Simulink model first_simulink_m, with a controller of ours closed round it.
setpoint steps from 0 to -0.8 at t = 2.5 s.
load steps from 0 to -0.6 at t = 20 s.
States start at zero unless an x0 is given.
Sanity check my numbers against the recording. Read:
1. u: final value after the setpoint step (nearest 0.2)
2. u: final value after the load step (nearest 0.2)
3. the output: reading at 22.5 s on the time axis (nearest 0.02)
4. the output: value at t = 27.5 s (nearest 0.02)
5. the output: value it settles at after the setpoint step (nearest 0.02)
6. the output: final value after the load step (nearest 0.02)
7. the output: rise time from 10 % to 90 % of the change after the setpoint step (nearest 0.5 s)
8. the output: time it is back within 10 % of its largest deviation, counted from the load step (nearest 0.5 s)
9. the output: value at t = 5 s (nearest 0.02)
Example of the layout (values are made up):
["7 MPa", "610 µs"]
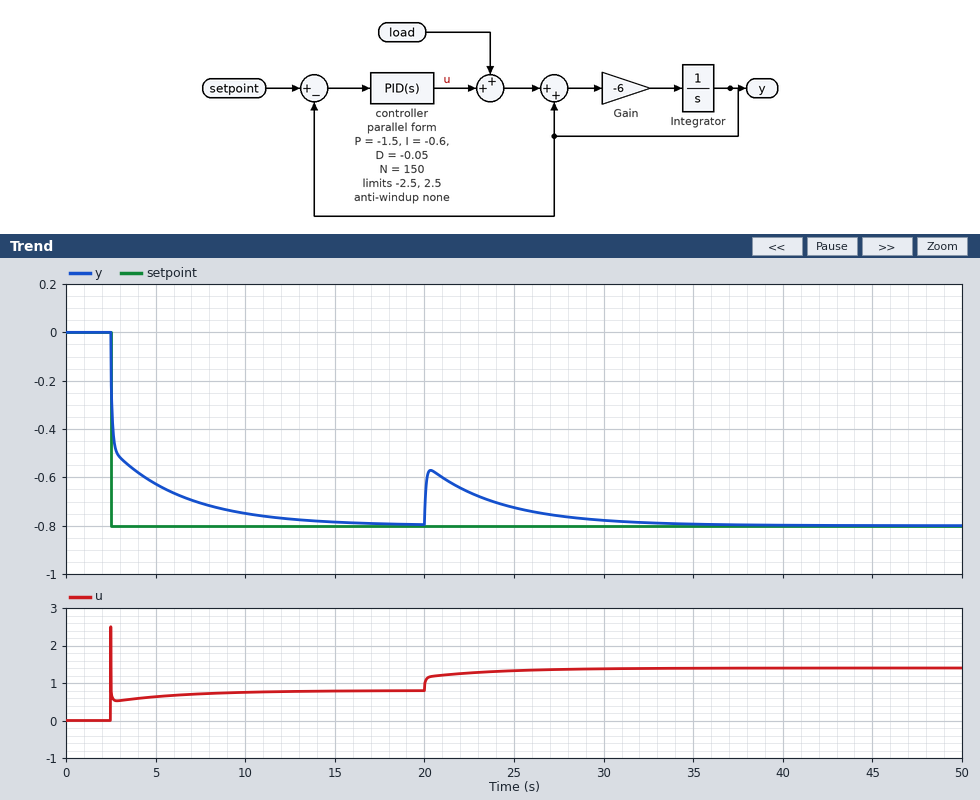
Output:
["0.8", "1.4", "-0.66", "-0.76", "-0.80", "-0.80", "5.5 s", "10.0 s", "-0.62"]
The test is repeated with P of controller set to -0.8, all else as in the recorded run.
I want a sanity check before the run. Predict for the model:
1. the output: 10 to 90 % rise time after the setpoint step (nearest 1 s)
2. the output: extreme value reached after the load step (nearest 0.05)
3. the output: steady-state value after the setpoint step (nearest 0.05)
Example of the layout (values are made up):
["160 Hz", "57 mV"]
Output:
["5 s", "-0.50", "-0.80"]
